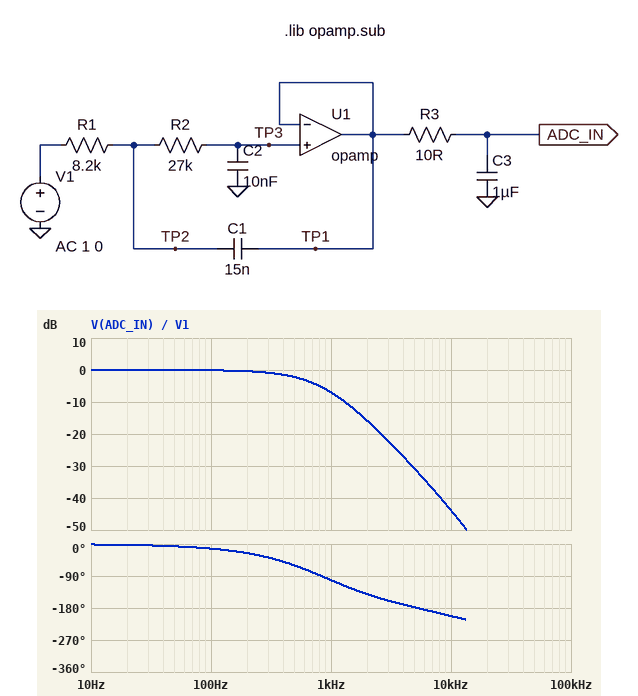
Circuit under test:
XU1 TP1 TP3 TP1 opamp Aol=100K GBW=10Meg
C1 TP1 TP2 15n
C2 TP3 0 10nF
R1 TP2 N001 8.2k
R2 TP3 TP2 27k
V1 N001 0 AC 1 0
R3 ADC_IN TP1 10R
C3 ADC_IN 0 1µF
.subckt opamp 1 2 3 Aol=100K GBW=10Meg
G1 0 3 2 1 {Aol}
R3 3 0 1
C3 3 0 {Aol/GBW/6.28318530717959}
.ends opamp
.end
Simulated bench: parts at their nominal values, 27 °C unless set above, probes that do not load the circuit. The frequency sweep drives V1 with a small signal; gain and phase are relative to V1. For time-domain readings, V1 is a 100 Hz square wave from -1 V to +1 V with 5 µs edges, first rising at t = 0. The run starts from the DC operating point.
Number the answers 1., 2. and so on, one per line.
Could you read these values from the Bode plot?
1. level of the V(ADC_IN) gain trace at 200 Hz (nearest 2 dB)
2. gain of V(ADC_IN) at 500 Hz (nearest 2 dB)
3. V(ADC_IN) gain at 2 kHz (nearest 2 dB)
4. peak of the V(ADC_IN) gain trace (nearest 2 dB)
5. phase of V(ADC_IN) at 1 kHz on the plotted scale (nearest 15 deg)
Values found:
1. 0 dB
2. -2 dB
3. -16 dB
4. 0 dB
5. -105 deg
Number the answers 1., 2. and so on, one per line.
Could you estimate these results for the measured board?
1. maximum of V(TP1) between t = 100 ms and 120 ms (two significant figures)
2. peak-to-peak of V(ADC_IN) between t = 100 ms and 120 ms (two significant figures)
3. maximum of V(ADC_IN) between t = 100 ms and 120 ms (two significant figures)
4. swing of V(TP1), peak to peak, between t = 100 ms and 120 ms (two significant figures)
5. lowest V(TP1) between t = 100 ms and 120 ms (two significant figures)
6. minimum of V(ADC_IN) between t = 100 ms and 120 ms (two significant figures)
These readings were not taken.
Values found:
1. 1.0 V
2. 2.0 V
3. 1.0 V
4. 2.0 V
5. -1.0 V
6. -1.0 V
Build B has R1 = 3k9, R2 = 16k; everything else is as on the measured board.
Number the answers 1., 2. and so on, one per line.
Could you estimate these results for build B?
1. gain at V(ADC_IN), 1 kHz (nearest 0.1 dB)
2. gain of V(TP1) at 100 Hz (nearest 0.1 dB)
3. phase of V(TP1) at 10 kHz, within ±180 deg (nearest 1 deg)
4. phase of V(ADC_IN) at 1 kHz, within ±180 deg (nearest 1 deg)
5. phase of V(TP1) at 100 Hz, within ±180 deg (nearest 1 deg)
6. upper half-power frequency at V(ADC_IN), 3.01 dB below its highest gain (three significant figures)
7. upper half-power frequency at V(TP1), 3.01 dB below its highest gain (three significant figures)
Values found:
1. -2.9 dB
2. 0 dB
3. -161 deg
4. -67 deg
5. -7 deg
6. 1.01 kHz
7. 1.02 kHz
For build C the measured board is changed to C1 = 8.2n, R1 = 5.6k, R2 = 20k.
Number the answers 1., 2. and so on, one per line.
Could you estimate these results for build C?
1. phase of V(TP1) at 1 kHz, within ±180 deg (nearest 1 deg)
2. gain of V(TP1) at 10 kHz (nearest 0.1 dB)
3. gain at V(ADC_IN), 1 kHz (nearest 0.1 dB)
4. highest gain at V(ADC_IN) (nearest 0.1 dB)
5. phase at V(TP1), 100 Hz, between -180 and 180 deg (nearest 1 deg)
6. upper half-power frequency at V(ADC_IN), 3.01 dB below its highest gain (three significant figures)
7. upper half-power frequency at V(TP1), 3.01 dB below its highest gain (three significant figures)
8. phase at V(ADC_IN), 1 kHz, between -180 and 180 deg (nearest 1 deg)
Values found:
1. -68 deg
2. -31.8 dB
3. -4.8 dB
4. 0 dB
5. -9 deg
6. 718 Hz
7. 720 Hz
8. -72 deg
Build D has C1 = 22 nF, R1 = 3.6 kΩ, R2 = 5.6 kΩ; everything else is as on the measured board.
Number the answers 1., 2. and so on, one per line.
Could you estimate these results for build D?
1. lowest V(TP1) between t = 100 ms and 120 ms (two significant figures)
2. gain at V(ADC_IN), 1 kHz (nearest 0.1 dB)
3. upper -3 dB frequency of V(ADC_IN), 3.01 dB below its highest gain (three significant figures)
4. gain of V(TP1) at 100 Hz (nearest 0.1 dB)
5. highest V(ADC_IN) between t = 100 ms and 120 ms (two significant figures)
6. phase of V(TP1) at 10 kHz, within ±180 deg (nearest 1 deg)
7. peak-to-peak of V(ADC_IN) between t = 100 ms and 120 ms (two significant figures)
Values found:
1. -1.1 V
2. -0.1 dB
3. 2.42 kHz
4. 0 dB
5. 1.1 V
6. -161 deg
7. 2.2 V
